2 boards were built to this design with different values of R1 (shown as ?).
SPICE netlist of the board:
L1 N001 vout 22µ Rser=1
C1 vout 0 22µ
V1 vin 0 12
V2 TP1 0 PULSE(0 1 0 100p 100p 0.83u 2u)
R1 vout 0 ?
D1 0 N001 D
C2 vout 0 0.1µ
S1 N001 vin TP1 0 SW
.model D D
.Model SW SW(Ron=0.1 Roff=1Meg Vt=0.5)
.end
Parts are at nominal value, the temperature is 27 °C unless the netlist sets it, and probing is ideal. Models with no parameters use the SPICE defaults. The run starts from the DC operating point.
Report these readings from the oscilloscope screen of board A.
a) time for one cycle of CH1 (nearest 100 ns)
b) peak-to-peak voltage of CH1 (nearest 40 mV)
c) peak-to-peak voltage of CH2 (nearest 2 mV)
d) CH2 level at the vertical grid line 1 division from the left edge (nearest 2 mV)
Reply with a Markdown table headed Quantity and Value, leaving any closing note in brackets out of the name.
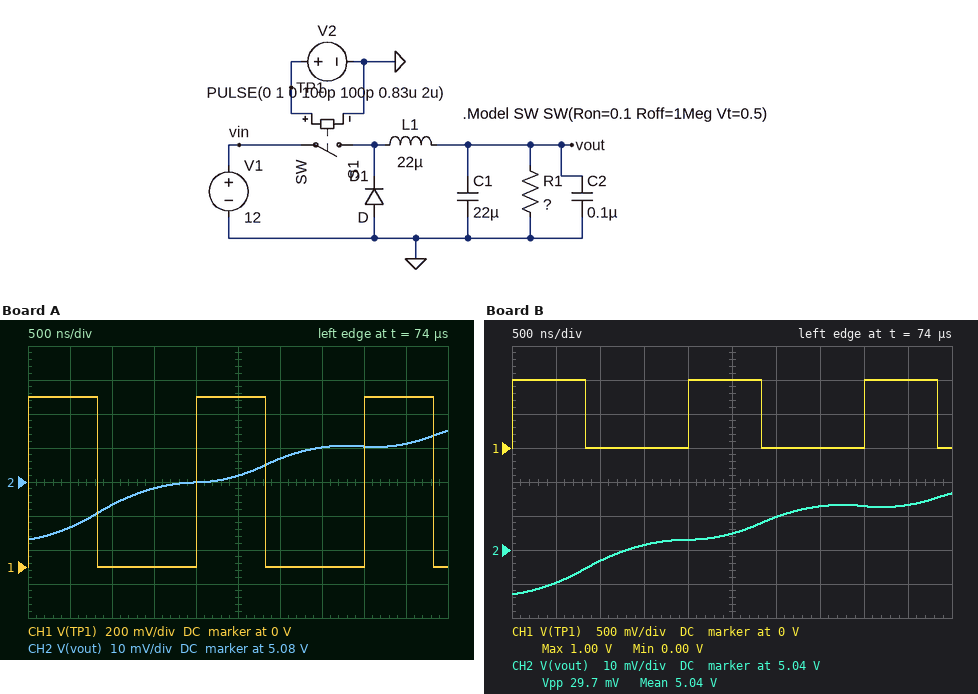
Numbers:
| Quantity | Value |
|---|---|
| time for one cycle of CH1 | 2.0 µs |
| peak-to-peak voltage of CH1 | 1.00 V |
| peak-to-peak voltage of CH2 | 32 mV |
| CH2 level at the vertical grid line 1 division from the left edge | 5.066 V |
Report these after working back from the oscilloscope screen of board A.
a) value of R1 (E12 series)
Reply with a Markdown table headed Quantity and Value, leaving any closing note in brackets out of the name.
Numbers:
| Quantity | Value |
|---|---|
| value of R1 | 120 Ω |
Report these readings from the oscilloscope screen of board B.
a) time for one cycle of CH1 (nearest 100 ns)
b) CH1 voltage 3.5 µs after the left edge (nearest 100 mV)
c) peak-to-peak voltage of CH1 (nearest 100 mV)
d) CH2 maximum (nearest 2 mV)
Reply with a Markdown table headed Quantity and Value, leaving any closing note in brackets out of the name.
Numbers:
| Quantity | Value |
|---|---|
| time for one cycle of CH1 | 2.0 µs |
| CH1 voltage 3.5 µs after the left edge | 0 V |
| peak-to-peak voltage of CH1 | 1.0 V |
| CH2 maximum | 5.056 V |
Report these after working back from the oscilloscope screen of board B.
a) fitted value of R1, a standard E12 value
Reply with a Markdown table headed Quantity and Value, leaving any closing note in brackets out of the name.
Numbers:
| Quantity | Value |
|---|---|
| fitted value of R1, a standard E12 value | 68 Ω |
